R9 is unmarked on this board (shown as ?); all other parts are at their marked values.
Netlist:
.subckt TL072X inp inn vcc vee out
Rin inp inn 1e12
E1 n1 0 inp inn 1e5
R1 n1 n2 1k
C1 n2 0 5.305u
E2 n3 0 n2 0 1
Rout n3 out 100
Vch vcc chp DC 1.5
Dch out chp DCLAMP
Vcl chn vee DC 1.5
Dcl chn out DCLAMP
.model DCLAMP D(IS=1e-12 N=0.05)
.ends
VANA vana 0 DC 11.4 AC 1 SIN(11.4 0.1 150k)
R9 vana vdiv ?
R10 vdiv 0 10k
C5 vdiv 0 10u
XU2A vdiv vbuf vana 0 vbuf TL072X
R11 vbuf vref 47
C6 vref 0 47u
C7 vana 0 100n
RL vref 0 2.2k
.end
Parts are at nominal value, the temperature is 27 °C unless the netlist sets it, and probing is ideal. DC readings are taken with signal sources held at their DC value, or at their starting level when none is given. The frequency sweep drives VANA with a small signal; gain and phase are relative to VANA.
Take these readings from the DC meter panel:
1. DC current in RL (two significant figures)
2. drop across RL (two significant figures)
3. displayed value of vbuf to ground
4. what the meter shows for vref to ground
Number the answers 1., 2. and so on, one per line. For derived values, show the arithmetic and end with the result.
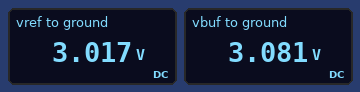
1. (3.017 V) / 2.2 kΩ = 1.4 mA
2. 3.017 V = 3.0 V
3. 3.081 V
4. 3.017 V
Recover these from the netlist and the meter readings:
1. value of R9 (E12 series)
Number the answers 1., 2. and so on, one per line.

1. 27 kΩ
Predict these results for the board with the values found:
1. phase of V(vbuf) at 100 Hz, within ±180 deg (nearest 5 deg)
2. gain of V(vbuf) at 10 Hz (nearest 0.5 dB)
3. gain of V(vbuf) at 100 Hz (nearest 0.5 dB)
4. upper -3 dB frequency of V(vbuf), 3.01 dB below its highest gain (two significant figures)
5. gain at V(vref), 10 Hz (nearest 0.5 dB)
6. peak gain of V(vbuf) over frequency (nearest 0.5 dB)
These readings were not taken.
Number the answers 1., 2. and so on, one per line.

1. -90 deg
2. -25.0 dB
3. -44.5 dB
4. 2.2 Hz
5. -25.0 dB
6. -11.5 dB
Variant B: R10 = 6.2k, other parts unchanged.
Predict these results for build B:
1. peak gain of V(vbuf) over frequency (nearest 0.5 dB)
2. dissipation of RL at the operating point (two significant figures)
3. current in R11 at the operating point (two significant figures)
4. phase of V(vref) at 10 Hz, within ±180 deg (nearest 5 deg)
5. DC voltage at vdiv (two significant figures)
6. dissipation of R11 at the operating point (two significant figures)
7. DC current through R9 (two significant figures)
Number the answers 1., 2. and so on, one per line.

1. -14.5 dB
2. 2.0 mW
3. 950 µA
4. -80 deg
5. 2.1 V
6. 42 µW
7. 340 µA
